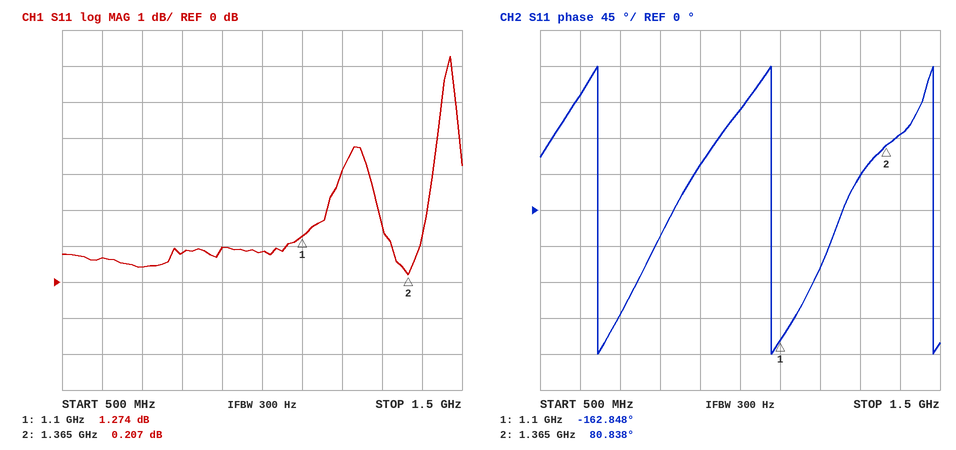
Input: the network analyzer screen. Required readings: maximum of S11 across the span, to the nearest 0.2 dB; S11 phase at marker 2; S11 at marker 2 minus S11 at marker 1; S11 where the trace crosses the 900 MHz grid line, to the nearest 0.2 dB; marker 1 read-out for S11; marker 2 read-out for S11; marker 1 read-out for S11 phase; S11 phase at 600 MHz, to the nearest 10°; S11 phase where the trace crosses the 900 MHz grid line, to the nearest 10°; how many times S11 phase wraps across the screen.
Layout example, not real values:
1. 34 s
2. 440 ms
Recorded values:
1. 6.2 dB
2. 80.838°
3. -1.067 dB
4. 1.0 dB
5. 1.274 dB
6. 0.207 dB
7. -162.848°
8. 140°
9. 60°
10. 3
